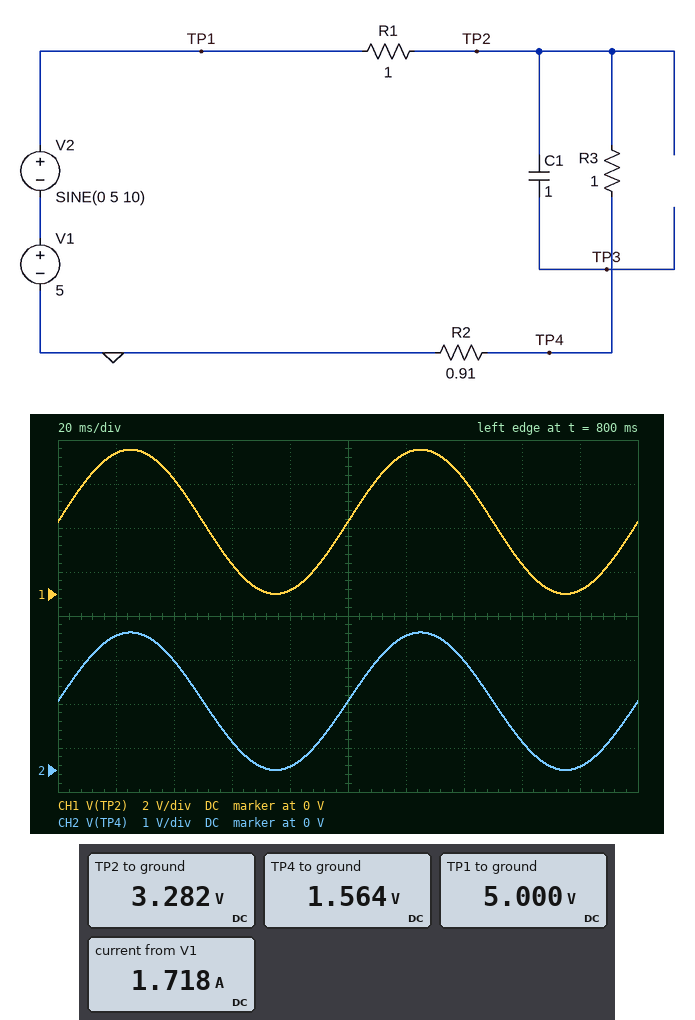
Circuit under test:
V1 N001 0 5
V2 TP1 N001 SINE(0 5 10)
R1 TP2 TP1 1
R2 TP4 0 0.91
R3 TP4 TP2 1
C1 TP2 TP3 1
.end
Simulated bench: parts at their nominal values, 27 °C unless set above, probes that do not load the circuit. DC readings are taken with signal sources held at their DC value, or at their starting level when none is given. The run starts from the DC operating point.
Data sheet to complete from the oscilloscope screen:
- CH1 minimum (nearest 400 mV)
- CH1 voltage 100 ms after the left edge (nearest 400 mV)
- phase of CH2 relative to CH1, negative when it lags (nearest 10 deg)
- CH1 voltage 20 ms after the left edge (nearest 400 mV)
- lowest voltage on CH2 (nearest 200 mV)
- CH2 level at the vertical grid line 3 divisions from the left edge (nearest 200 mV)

0 V
3.2 V
0 deg
6.4 V
0 V
600 mV
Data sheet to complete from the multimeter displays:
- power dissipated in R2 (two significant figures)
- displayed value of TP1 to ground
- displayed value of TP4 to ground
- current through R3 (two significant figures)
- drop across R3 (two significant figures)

2.7 W
5.000 V
1.564 V
1.7 A
1.7 V
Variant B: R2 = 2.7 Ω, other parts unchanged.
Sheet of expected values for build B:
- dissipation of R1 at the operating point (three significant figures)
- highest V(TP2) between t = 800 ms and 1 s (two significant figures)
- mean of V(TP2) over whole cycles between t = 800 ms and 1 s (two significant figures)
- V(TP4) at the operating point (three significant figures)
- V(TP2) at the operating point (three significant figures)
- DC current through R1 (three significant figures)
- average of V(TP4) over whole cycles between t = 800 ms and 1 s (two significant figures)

1.13 W
7.9 V
3.9 V
2.87 V
3.94 V
1.06 A
2.9 V
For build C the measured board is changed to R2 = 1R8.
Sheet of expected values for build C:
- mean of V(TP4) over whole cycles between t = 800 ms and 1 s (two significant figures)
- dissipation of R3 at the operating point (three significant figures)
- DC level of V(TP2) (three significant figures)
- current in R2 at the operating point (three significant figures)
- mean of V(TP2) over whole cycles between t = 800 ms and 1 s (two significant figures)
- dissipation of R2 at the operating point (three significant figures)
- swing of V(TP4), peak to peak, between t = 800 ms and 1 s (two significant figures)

2.4 V
1.73 W
3.68 V
1.32 A
3.7 V
3.12 W
4.7 V
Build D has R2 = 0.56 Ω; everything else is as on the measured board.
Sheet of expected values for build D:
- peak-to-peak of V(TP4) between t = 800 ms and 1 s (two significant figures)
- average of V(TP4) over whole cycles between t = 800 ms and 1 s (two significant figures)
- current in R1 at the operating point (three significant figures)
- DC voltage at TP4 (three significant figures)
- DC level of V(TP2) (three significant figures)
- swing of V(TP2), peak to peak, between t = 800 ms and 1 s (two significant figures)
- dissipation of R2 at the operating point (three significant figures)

2.2 V
1.1 V
1.95 A
1.09 V
3.05 V
6.1 V
2.14 W
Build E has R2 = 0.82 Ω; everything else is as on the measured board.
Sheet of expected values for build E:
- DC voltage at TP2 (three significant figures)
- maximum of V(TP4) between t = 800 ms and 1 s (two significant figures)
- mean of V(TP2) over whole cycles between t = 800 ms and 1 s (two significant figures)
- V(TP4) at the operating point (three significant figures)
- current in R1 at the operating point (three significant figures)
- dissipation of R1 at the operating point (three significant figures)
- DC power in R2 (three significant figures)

3.23 V
2.9 V
3.2 V
1.45 V
1.77 A
3.14 W
2.58 W
